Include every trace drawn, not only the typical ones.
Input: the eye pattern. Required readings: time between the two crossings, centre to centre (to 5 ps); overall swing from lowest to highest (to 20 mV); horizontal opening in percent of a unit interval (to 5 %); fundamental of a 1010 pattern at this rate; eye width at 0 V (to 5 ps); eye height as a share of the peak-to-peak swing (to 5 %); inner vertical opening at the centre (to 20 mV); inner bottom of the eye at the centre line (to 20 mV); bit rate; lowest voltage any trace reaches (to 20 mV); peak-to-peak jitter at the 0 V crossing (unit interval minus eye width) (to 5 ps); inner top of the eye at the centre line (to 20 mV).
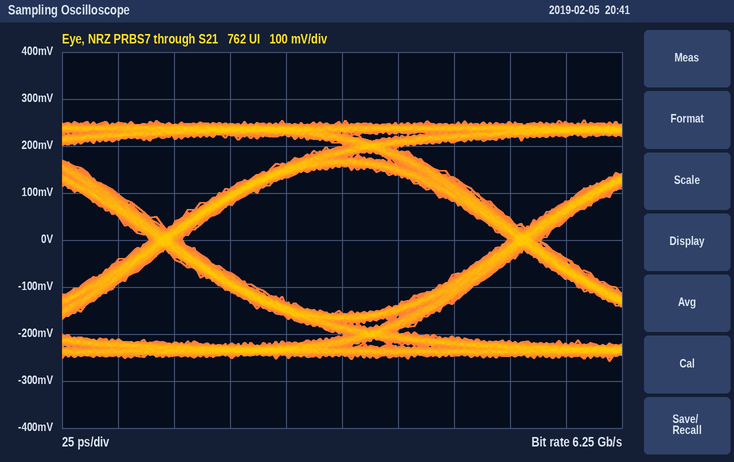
160 ps
520 mV
90 %
3.125 GHz
145 ps
60 %
320 mV
-160 mV
6.25 Gb/s
-260 mV
15 ps
160 mV
